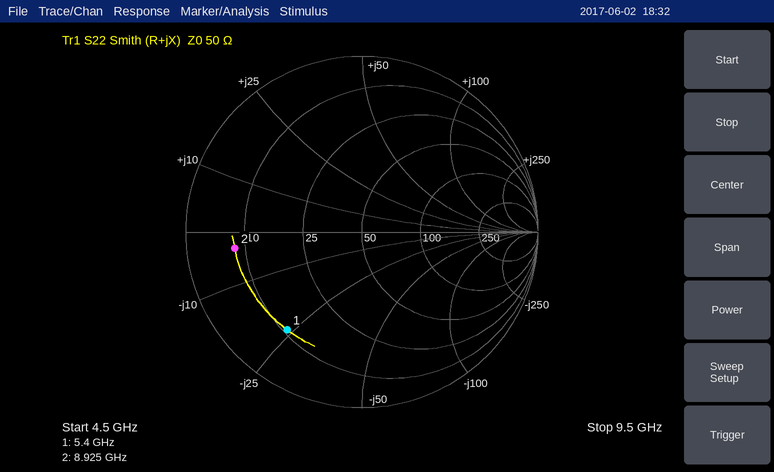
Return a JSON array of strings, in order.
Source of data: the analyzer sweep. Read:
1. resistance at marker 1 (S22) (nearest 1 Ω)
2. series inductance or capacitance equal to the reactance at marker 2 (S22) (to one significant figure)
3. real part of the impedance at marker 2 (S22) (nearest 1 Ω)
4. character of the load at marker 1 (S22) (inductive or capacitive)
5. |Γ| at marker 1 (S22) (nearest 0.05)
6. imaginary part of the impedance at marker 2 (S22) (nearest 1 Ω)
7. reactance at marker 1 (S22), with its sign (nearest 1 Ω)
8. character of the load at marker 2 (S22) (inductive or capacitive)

["11 Ω", "6 pF", "8 Ω", "capacitive", "0.70", "-3 Ω", "-24 Ω", "capacitive"]
